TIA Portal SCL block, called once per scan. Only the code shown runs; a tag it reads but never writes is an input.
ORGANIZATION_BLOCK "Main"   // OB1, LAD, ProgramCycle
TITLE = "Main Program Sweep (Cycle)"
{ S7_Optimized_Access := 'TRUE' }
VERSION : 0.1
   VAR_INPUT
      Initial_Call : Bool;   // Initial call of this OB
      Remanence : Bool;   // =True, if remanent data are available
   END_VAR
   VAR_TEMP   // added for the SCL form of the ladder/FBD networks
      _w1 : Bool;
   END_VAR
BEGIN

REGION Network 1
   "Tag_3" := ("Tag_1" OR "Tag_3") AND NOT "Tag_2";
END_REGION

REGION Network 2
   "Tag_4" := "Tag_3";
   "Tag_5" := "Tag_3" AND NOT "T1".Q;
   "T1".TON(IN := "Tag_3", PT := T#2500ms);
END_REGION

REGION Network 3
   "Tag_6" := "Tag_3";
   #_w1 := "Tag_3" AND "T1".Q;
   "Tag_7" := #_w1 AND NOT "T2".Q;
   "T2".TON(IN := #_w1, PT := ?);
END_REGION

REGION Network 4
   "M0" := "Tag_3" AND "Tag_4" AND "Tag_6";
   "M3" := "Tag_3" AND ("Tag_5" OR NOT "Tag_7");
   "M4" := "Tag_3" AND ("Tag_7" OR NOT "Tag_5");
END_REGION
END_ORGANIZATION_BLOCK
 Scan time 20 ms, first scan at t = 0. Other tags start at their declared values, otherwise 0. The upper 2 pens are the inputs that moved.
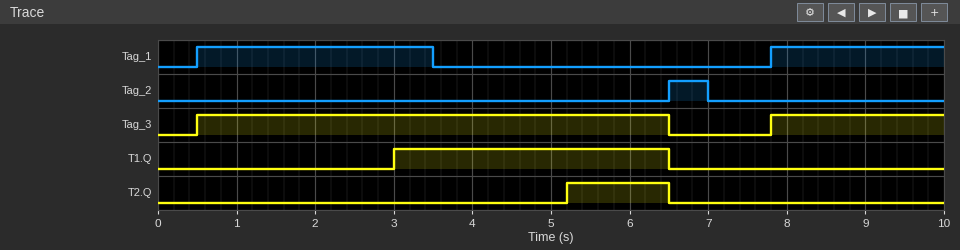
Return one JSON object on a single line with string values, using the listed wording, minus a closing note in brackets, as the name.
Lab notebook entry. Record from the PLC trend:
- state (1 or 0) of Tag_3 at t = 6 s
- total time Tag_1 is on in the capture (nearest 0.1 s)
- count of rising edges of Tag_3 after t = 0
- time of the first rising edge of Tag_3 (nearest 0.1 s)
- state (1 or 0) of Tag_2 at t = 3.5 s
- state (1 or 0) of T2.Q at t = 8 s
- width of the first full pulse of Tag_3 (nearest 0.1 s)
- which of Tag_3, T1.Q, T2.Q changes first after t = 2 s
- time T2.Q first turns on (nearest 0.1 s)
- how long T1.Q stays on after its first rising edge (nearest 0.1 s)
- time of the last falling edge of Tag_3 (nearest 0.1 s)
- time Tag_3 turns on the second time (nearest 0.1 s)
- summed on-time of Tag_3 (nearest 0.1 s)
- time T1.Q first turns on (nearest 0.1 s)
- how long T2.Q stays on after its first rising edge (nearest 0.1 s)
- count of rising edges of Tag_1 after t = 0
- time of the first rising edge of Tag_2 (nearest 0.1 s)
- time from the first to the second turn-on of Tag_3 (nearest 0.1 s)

{"state (1 or 0) of Tag_3 at t = 6 s": "1", "total time Tag_1 is on in the capture": "5.2 s", "count of rising edges of Tag_3 after t = 0": "2", "time of the first rising edge of Tag_3": "0.5 s", "state (1 or 0) of Tag_2 at t = 3.5 s": "0", "state (1 or 0) of T2.Q at t = 8 s": "0", "width of the first full pulse of Tag_3": "6.0 s", "which of Tag_3, T1.Q, T2.Q changes first after t = 2 s": "T1.Q", "time T2.Q first turns on": "5.2 s", "how long T1.Q stays on after its first rising edge": "3.5 s", "time of the last falling edge of Tag_3": "6.5 s", "time Tag_3 turns on the second time": "7.8 s", "summed on-time of Tag_3": "8.2 s", "time T1.Q first turns on": "3.0 s", "how long T2.Q stays on after its first rising edge": "1.3 s", "count of rising edges of Tag_1 after t = 0": "2", "time of the first rising edge of Tag_2": "6.5 s", "time from the first to the second turn-on of Tag_3": "7.3 s"}
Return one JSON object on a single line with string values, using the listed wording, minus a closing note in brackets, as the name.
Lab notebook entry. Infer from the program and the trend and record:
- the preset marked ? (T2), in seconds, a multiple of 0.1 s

{"the preset marked ? (T2), in seconds, a multiple of 0.1 s": "2.2 s"}
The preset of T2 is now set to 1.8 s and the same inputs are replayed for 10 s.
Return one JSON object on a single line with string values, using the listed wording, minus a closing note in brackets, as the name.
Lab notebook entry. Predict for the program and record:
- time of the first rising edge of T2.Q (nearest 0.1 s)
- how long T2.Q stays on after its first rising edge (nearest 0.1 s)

{"time of the first rising edge of T2.Q": "4.8 s", "how long T2.Q stays on after its first rising edge": "1.7 s"}
